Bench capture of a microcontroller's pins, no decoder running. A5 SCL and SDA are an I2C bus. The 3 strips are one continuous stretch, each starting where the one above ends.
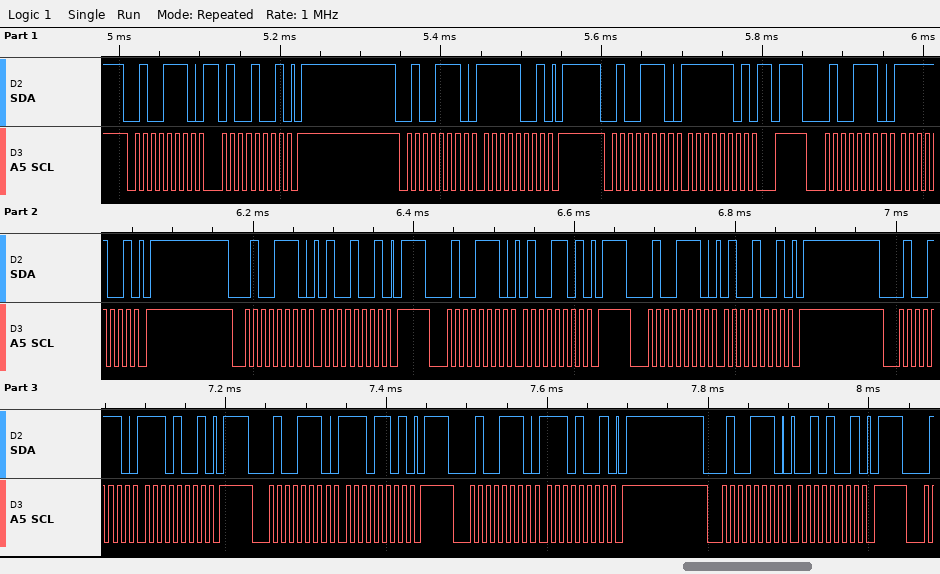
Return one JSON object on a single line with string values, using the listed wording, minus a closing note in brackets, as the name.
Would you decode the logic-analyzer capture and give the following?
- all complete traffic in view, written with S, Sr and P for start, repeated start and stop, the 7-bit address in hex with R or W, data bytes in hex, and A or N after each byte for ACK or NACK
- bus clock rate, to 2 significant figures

{"all complete traffic in view, written with S, Sr and P for start, repeated start and stop, the 7-bit address in hex with R or W, data bytes in hex, and A or N after each byte for ACK or NACK": "S 27W A 49 A P S 27W A F9 A P S 27W A FD A P S 27W A F9 A P S 27W A 49 A P S 27W A 4D A P S 27W A 49 A P S 27W A E9 A P S 27W A ED A P S 27W A E9 A P S 27W A 29 A P", "bus clock rate, to 2 significant figures": "100 kHz"}
